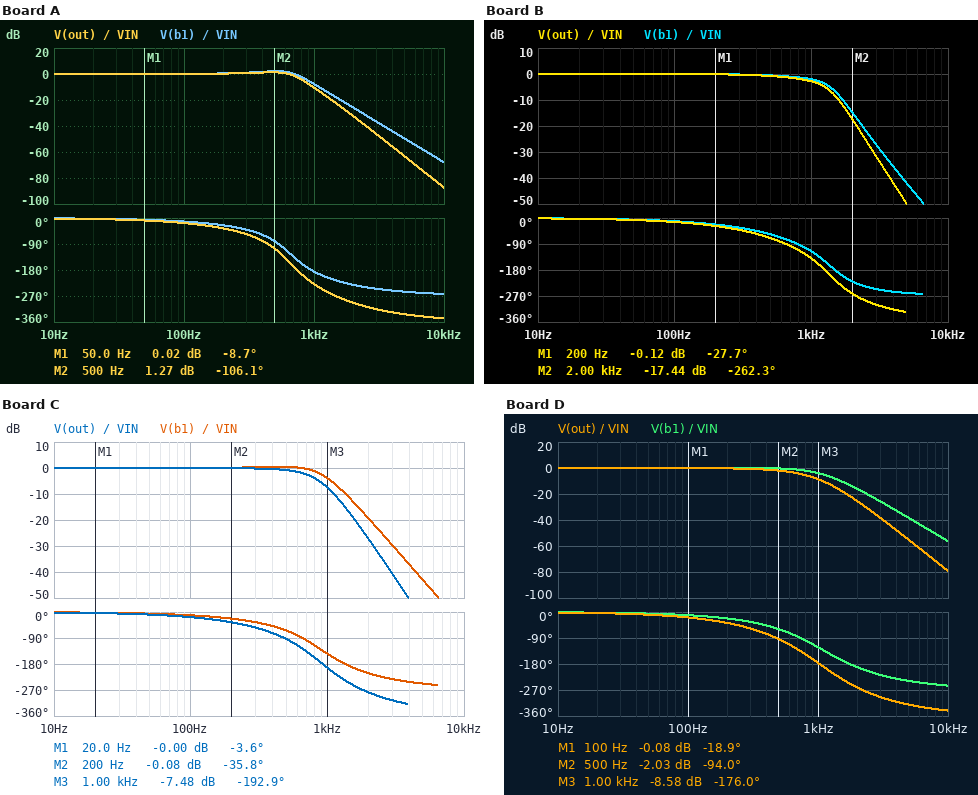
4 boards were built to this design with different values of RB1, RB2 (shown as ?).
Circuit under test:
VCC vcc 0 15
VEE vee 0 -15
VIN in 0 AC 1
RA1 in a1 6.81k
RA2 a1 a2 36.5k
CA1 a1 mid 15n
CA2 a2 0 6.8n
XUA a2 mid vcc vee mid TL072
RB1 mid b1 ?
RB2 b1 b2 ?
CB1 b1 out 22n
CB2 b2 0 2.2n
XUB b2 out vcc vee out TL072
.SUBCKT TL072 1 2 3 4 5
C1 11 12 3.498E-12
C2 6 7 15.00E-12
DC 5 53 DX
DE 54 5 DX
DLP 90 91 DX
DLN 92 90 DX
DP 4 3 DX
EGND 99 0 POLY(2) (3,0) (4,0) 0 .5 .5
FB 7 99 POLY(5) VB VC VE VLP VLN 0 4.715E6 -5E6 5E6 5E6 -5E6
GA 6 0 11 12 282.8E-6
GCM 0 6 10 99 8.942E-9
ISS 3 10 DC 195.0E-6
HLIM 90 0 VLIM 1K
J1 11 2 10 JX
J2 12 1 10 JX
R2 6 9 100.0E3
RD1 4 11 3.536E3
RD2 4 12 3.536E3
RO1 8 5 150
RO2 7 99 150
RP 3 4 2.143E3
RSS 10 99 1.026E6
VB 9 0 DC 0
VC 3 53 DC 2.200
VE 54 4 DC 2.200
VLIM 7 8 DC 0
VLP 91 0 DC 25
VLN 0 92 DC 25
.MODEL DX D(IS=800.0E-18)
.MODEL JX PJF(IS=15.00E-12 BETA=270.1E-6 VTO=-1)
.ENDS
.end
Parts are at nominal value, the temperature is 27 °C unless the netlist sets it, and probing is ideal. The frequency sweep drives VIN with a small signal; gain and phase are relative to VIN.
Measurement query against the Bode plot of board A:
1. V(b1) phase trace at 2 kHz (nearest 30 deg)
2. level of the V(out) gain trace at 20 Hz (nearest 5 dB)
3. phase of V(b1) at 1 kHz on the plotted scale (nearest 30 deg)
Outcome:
-240 deg
0 dB
-180 deg
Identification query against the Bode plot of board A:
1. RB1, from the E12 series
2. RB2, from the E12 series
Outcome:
18 kΩ
68 kΩ
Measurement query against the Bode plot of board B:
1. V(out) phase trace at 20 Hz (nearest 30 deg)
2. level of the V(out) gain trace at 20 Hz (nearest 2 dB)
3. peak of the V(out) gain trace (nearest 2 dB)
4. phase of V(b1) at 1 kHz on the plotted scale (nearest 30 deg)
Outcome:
0 deg
0 dB
0 dB
-120 deg
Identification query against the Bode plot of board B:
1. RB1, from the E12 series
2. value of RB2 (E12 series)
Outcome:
8.2 kΩ
33 kΩ
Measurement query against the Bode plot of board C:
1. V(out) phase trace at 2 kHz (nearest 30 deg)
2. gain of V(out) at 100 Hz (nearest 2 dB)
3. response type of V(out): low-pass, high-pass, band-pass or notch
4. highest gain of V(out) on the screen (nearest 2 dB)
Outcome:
-270 deg
0 dB
low-pass
0 dB
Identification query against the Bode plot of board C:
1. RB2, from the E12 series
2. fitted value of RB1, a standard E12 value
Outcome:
82 kΩ
8.2 kΩ
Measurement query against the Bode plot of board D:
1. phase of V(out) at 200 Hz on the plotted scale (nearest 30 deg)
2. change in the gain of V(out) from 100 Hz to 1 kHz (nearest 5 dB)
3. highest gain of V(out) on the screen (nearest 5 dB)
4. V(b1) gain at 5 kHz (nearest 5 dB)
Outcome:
-30 deg
-10 dB
0 dB
-40 dB
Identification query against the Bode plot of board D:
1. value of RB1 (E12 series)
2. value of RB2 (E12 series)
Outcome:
4.7 kΩ
100 kΩ
